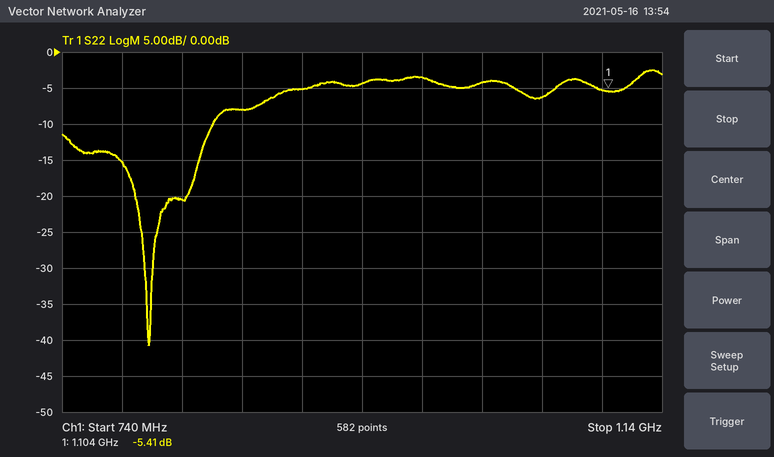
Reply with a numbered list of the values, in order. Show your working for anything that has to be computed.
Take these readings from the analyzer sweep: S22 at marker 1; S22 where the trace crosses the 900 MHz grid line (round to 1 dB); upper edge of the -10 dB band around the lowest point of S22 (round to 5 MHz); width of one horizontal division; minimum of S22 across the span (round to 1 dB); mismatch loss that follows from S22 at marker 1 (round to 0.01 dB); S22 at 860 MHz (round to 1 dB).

1. -5.41 dB
2. -5 dB
3. 840 MHz
4. 40 MHz
5. -41 dB
6. −10 log10(1 − 10^(-5.41/10)) ≈ 1.47 dB
7. -8 dB
